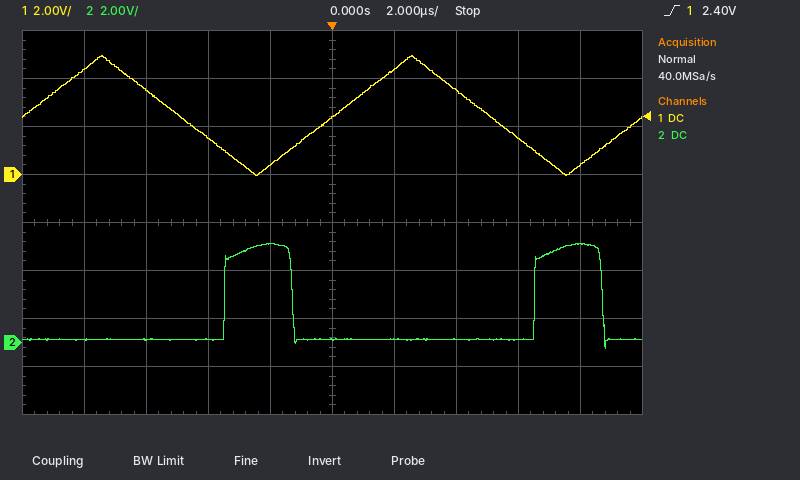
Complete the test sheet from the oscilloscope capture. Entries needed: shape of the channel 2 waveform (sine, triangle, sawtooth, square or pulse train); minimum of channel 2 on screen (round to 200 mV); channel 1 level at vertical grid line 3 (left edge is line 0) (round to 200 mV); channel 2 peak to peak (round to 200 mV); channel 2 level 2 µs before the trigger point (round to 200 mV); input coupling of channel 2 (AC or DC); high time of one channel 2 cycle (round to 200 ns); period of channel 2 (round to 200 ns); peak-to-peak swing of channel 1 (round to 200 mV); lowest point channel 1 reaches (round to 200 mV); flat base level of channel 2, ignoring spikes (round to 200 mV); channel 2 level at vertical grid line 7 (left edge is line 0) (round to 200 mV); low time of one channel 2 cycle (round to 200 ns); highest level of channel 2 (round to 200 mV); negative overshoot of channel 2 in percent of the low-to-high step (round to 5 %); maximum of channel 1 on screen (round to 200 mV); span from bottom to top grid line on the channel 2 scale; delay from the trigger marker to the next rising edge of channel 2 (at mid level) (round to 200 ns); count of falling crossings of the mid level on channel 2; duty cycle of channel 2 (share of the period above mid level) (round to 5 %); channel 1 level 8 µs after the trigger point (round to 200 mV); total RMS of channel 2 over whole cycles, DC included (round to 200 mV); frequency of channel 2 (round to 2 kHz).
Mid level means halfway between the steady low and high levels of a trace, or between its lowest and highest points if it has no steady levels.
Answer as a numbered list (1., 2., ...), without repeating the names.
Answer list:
1. pulse train
2. -200 mV
3. 1.6 V
4. 4.4 V
5. 4.2 V
6. DC
7. 2.2 µs
8. 10.0 µs
9. 5.0 V
10. 0.0 V
11. 200 mV
12. 200 mV
13. 7.8 µs
14. 4.2 V
15. 10 %
16. 5.0 V
17. 16 V
18. 6.6 µs
19. 2
20. 20 %
21. 400 mV
22. 1.8 V
23. 100 kHz
